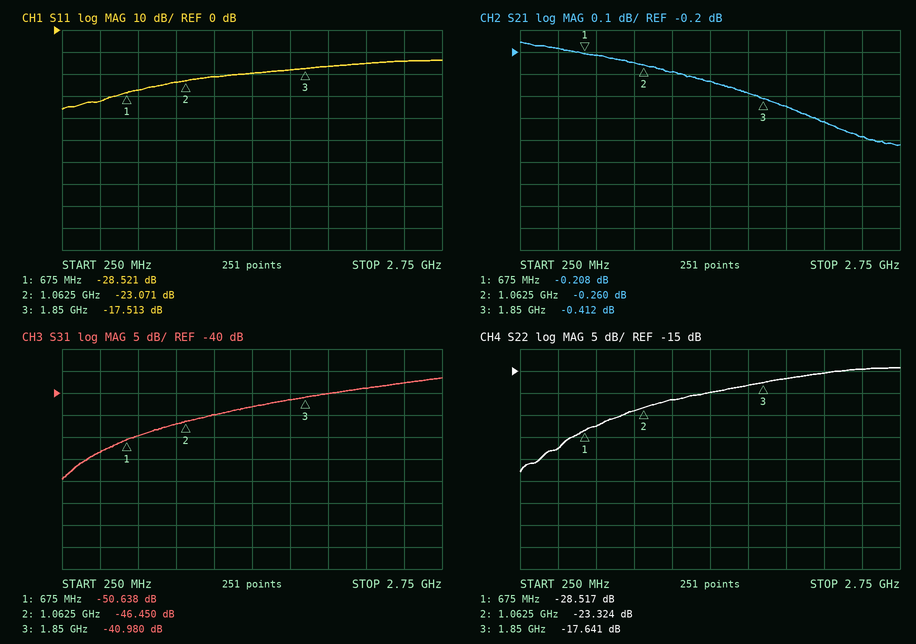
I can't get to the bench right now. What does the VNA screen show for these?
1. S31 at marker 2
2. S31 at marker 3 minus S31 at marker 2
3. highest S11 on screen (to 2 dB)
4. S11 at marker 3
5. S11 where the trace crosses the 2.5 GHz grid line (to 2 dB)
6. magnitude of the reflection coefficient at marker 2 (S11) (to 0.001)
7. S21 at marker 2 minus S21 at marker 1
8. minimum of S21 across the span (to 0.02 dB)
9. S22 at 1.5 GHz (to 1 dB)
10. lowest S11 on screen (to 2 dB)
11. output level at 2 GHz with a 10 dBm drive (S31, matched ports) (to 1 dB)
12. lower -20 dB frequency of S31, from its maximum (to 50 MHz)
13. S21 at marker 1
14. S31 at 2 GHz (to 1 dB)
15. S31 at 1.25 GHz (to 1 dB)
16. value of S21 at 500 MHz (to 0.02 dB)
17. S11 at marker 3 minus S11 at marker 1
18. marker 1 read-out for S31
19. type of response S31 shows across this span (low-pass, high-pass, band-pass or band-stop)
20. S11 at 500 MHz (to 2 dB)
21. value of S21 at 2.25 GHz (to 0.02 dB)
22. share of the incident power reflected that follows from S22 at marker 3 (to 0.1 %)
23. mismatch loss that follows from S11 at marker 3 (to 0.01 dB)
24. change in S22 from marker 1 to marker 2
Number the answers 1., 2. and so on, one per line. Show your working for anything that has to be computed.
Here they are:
1. -46.450 dB
2. -40.98 − (-46.45) = 5.470 dB
3. -14 dB
4. -17.513 dB
5. -14 dB
6. 10^(-23.071/20) ≈ 0.070
7. -0.26 − (-0.208) = -0.052 dB
8. -0.62 dB
9. -20 dB
10. -36 dB
11. 10 dBm + (-40 dB) = -30 dBm
12. 350 MHz
13. -0.208 dB
14. -40 dB
15. -45 dB
16. -0.18 dB
17. -17.513 − (-28.521) = 11.008 dB
18. -50.638 dB
19. high-pass
20. -32 dB
21. -0.52 dB
22. 10^(-17.641/10) ≈ 1.7 %
23. −10 log10(1 − 10^(-17.513/10)) ≈ 0.08 dB
24. -23.324 − (-28.517) = 5.193 dB
